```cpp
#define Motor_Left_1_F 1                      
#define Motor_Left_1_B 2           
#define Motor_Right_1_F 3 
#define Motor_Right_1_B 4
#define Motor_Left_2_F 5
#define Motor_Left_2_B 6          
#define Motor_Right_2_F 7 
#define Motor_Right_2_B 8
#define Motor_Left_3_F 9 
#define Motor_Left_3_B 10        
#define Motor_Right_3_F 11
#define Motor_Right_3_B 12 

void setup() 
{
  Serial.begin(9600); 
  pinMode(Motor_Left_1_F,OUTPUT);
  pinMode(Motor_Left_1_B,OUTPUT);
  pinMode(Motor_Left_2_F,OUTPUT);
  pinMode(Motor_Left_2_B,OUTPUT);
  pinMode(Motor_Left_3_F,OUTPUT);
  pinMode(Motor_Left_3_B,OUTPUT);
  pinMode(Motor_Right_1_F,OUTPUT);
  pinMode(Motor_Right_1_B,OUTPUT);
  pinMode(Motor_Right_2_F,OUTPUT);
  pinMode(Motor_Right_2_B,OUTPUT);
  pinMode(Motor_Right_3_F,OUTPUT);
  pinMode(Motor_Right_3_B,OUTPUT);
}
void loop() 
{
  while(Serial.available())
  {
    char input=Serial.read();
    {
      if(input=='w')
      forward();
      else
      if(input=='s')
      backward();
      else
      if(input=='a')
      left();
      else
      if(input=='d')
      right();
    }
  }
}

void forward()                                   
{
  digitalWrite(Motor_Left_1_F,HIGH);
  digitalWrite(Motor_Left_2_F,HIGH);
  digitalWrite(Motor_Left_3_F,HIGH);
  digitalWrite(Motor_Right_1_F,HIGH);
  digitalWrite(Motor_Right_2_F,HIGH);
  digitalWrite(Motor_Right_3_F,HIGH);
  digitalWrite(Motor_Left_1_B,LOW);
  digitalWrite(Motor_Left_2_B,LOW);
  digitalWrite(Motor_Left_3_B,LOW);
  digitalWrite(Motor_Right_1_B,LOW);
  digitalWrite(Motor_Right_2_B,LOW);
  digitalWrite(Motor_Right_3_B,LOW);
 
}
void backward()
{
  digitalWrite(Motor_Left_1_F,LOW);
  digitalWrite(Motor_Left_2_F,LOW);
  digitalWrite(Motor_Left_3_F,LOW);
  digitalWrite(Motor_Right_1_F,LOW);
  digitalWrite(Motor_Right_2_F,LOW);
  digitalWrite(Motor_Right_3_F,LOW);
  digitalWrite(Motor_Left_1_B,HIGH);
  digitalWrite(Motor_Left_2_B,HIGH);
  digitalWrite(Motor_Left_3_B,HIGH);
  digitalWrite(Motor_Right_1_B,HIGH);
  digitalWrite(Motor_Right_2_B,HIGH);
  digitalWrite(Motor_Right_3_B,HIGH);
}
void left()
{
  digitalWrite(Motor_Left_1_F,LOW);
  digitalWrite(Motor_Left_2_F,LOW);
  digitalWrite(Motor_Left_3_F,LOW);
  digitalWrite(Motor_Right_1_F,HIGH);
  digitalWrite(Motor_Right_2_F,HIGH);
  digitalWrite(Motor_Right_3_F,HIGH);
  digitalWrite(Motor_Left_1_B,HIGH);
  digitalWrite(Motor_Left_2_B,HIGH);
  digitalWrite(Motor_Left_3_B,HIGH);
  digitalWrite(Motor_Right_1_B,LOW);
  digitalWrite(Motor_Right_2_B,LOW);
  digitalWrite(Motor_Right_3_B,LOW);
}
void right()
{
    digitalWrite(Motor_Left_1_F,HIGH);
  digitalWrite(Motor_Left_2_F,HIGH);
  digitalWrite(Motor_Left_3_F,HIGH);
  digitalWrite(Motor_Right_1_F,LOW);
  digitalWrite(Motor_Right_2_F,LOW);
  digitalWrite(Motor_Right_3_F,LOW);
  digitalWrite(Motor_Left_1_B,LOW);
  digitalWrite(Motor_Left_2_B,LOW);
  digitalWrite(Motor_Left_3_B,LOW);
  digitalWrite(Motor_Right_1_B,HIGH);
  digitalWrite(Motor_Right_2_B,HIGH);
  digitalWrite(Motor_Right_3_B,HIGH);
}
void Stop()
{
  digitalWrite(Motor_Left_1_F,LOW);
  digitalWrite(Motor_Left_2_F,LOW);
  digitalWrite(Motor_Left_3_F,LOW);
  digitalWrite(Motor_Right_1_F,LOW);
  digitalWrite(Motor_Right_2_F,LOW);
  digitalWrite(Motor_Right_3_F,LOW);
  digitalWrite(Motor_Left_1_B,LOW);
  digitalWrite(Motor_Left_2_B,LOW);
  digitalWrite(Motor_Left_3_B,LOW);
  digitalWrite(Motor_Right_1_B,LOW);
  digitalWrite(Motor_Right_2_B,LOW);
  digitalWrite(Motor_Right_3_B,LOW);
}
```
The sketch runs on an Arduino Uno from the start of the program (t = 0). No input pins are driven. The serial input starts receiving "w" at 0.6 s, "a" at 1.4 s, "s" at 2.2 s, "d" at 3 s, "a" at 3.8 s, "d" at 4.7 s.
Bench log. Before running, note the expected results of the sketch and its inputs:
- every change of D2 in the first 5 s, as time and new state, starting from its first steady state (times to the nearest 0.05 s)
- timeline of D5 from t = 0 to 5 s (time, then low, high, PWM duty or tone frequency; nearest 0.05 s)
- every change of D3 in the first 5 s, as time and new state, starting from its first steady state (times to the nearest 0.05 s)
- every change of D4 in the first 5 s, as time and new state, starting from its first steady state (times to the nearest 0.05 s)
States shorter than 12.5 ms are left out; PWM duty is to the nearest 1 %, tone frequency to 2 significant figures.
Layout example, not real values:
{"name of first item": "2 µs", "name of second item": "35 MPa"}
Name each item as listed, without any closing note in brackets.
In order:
{"every change of D2 in the first 5 s, as time and new state, starting from its first steady state": "0 s low; 1.4 s high; 3 s low; 3.8 s high; 4.7 s low", "timeline of D5 from t = 0 to 5 s": "0 s low; 0.6 s high; 1.4 s low; 3 s high; 3.8 s low; 4.7 s high", "every change of D3 in the first 5 s, as time and new state, starting from its first steady state": "0 s low; 0.6 s high; 2.2 s low; 3.8 s high; 4.7 s low", "every change of D4 in the first 5 s, as time and new state, starting from its first steady state": "0 s low; 2.2 s high; 3.8 s low; 4.7 s high"}
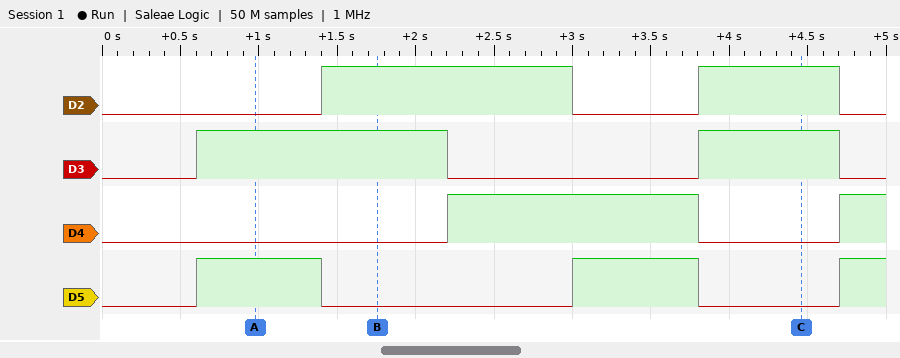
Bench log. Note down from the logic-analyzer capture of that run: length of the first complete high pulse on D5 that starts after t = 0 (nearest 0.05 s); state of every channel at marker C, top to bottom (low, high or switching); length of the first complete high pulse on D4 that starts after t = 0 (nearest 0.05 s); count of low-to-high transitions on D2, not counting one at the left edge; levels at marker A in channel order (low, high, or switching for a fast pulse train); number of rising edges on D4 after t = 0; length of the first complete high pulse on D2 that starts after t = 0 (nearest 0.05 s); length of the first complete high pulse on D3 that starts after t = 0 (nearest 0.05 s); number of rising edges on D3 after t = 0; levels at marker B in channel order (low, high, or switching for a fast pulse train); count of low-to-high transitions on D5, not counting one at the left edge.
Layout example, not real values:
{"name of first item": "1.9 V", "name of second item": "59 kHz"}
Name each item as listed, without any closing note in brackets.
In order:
{"length of the first complete high pulse on D5 that starts after t = 0": "0.80 s", "state of every channel at marker C, top to bottom": "D2 high, D3 high, D4 low, D5 low", "length of the first complete high pulse on D4 that starts after t = 0": "1.60 s", "count of low-to-high transitions on D2, not counting one at the left edge": "2", "levels at marker A in channel order": "D2 low, D3 high, D4 low, D5 high", "number of rising edges on D4 after t = 0": "2", "length of the first complete high pulse on D2 that starts after t = 0": "1.60 s", "length of the first complete high pulse on D3 that starts after t = 0": "1.60 s", "number of rising edges on D3 after t = 0": "2", "levels at marker B in channel order": "D2 high, D3 high, D4 low, D5 low", "count of low-to-high transitions on D5, not counting one at the left edge": "3"}
